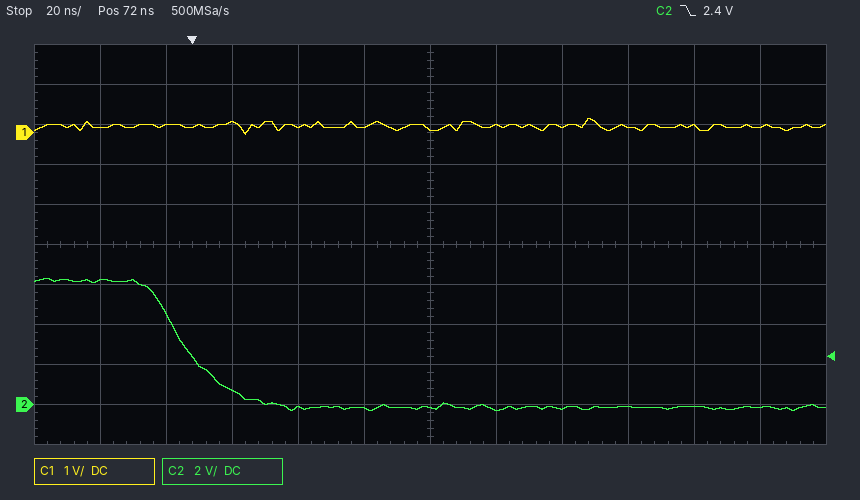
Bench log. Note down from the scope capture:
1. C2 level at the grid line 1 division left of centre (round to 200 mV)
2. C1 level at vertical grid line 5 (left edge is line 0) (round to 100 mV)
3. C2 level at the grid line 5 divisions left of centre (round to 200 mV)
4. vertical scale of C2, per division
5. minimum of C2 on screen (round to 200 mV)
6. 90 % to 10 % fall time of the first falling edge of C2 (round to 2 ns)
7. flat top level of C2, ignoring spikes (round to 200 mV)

-200 mV
100 mV
6.2 V
2 V
-400 mV
26 ns
6.2 V
